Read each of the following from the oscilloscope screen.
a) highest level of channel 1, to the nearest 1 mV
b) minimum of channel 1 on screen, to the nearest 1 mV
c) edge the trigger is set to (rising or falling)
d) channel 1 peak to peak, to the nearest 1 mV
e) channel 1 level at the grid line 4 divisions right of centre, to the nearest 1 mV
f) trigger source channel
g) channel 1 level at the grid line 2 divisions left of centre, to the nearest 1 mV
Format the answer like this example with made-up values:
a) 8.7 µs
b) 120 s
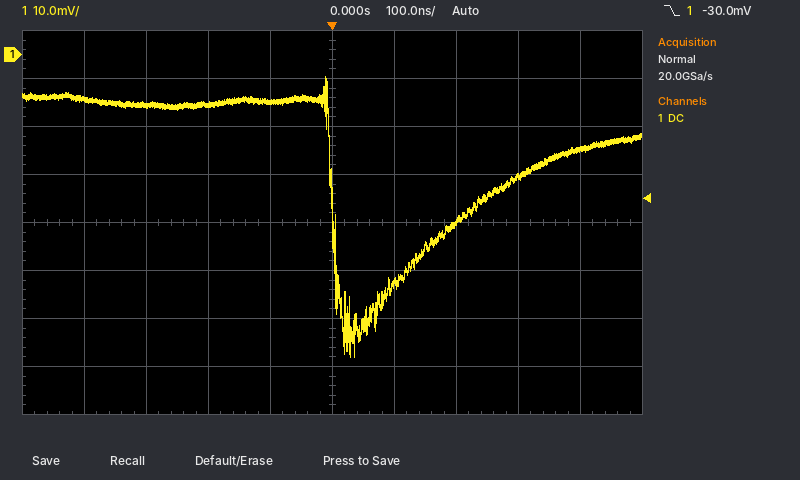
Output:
a) -5 mV
b) -63 mV
c) falling
d) 58 mV
e) -20 mV
f) channel 1
g) -10 mV
